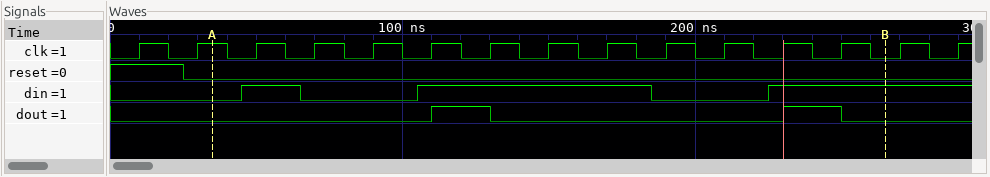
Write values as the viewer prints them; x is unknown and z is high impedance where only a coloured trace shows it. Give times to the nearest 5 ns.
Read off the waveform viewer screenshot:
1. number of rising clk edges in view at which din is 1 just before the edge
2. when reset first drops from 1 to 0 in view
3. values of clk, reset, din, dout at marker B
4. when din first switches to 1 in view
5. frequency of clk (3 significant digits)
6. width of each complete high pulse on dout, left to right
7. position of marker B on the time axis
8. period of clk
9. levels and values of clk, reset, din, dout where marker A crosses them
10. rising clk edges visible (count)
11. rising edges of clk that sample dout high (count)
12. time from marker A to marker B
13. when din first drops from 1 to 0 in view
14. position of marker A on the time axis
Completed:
9
25 ns
clk=0, reset=0, din=1, dout=0
45 ns
50.0 MHz
20 ns, 20 ns
265 ns
20 ns
clk=1, reset=0, din=0, dout=0
15
2
230 ns
65 ns
35 ns
